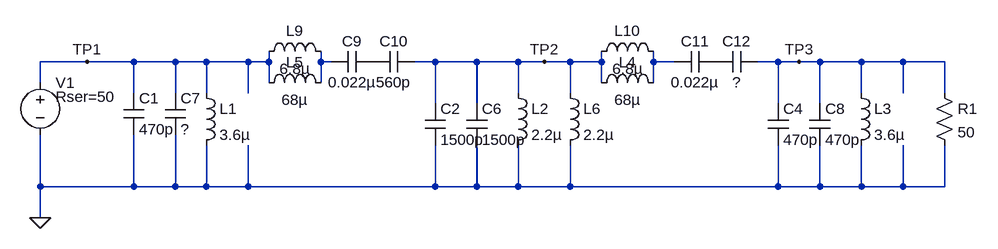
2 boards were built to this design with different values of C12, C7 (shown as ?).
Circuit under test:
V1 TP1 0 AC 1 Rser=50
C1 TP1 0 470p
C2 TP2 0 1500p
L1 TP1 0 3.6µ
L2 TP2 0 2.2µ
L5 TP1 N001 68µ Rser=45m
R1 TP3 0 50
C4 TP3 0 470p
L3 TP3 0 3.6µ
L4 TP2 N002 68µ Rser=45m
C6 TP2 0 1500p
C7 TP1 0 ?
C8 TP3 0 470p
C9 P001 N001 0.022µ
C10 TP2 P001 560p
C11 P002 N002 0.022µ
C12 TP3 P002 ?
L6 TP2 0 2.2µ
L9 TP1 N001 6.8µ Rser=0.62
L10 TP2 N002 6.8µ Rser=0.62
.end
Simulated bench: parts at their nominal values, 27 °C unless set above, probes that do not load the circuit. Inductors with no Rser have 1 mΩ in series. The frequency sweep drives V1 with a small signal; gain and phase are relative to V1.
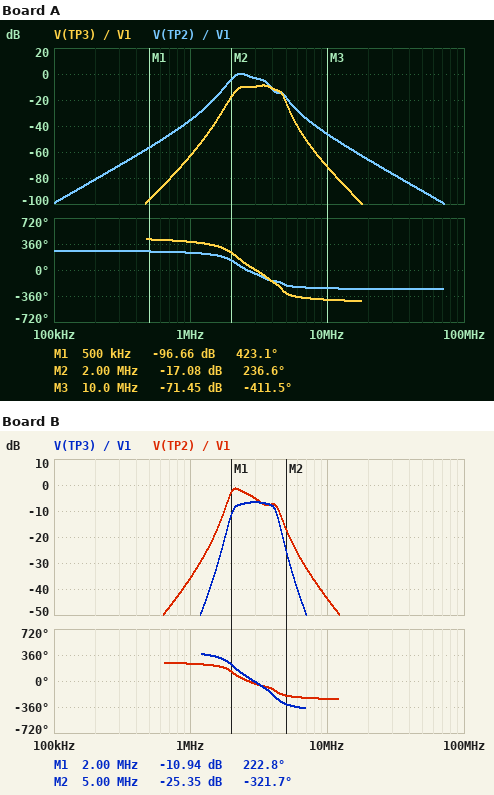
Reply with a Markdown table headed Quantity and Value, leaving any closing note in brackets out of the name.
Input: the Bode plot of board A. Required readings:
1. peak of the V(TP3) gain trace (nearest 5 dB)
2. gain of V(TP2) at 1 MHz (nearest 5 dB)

| Quantity | Value |
|---|---|
| peak of the V(TP3) gain trace | -10 dB |
| gain of V(TP2) at 1 MHz | -35 dB |
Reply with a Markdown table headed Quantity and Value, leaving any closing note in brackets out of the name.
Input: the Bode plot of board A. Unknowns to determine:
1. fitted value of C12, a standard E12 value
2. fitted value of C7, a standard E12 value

| Quantity | Value |
|---|---|
| fitted value of C12, a standard E12 value | 270 pF |
| fitted value of C7, a standard E12 value | 680 pF |
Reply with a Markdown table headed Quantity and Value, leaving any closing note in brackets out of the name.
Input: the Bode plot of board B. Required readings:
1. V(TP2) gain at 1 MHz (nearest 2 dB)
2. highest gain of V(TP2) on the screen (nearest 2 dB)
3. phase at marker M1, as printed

| Quantity | Value |
|---|---|
| V(TP2) gain at 1 MHz | -36 dB |
| highest gain of V(TP2) on the screen | -2 dB |
| phase at marker M1, as printed | 222.8 deg |
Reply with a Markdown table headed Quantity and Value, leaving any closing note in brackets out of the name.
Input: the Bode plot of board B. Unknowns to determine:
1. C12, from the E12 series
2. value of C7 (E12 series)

| Quantity | Value |
|---|---|
| C12, from the E12 series | 390 pF |
| value of C7 | 390 pF |
